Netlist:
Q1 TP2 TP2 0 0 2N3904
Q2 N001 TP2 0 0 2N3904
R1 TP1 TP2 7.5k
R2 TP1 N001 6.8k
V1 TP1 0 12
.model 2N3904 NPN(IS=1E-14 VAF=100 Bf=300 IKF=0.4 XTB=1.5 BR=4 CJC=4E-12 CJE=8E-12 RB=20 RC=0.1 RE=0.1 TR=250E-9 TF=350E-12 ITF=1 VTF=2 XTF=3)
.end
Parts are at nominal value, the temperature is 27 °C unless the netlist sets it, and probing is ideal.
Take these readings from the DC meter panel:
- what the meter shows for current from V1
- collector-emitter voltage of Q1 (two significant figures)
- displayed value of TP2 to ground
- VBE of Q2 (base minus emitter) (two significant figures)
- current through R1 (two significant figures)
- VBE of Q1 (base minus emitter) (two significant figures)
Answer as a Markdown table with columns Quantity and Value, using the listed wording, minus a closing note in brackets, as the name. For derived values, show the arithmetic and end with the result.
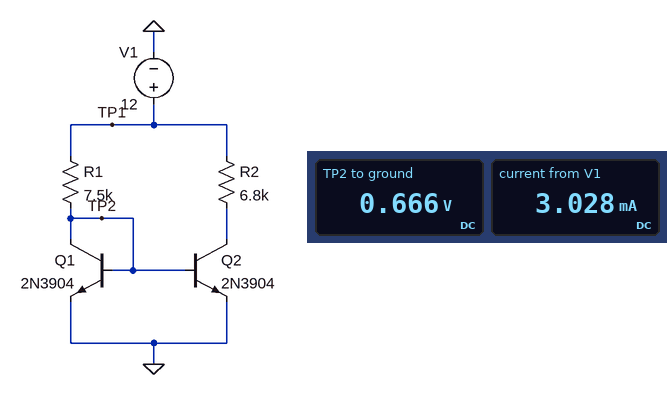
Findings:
| Quantity | Value |
|---|---|
| what the meter shows for current from V1 | 3.028 mA |
| collector-emitter voltage of Q1 | 666 mV = 670 mV |
| displayed value of TP2 to ground | 0.666 V |
| VBE of Q2 (base minus emitter) | 666 mV = 670 mV |
| current through R1 | (12 V - 666 mV) / 7.5 kΩ = 1.5 mA |
| VBE of Q1 (base minus emitter) | 666 mV = 670 mV |
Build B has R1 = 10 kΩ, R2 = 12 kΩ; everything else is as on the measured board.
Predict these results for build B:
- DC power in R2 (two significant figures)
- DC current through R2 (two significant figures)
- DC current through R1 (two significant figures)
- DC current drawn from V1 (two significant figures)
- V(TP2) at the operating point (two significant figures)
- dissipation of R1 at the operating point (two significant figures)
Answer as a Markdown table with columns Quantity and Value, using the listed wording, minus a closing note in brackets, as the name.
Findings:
| Quantity | Value |
|---|---|
| DC power in R2 | 12 mW |
| DC current through R2 | 990 µA |
| DC current through R1 | 1.1 mA |
| DC current drawn from V1 | 2.1 mA |
| V(TP2) at the operating point | 660 mV |
| dissipation of R1 at the operating point | 13 mW |
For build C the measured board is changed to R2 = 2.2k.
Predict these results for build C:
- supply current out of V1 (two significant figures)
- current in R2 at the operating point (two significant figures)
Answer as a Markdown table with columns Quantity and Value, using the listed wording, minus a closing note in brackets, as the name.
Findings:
| Quantity | Value |
|---|---|
| supply current out of V1 | 3.1 mA |
| current in R2 at the operating point | 1.6 mA |
